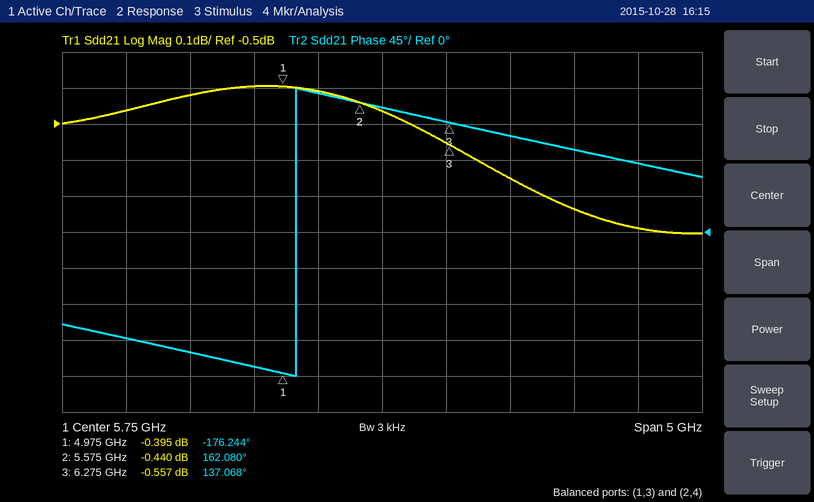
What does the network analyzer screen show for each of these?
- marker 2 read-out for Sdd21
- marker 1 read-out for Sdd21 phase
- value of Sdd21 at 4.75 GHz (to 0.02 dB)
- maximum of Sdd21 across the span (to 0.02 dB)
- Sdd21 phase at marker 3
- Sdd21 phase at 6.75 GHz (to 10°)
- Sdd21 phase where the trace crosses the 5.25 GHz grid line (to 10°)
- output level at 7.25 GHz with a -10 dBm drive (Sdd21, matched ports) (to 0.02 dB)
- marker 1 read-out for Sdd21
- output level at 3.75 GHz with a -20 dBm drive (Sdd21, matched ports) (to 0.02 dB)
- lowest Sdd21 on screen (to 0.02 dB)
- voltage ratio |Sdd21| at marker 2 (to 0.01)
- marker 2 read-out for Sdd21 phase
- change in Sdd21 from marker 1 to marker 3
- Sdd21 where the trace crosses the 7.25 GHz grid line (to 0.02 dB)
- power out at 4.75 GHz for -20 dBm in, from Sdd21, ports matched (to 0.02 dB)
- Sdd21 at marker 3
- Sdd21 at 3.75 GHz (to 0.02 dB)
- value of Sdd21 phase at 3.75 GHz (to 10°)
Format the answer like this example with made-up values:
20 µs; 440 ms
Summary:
-0.440 dB; -176.244°; -0.40 dB; -0.40 dB; 137.068°; 120°; 170°; -10.74 dBm; -0.395 dB; -20.46 dBm; -0.80 dB; 0.95; 162.080°; -0.162 dB; -0.74 dB; -20.40 dBm; -0.557 dB; -0.46 dB; -130°
